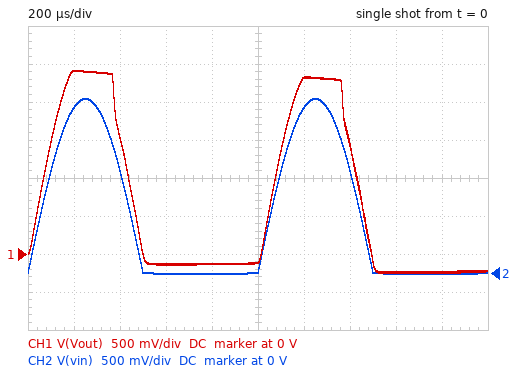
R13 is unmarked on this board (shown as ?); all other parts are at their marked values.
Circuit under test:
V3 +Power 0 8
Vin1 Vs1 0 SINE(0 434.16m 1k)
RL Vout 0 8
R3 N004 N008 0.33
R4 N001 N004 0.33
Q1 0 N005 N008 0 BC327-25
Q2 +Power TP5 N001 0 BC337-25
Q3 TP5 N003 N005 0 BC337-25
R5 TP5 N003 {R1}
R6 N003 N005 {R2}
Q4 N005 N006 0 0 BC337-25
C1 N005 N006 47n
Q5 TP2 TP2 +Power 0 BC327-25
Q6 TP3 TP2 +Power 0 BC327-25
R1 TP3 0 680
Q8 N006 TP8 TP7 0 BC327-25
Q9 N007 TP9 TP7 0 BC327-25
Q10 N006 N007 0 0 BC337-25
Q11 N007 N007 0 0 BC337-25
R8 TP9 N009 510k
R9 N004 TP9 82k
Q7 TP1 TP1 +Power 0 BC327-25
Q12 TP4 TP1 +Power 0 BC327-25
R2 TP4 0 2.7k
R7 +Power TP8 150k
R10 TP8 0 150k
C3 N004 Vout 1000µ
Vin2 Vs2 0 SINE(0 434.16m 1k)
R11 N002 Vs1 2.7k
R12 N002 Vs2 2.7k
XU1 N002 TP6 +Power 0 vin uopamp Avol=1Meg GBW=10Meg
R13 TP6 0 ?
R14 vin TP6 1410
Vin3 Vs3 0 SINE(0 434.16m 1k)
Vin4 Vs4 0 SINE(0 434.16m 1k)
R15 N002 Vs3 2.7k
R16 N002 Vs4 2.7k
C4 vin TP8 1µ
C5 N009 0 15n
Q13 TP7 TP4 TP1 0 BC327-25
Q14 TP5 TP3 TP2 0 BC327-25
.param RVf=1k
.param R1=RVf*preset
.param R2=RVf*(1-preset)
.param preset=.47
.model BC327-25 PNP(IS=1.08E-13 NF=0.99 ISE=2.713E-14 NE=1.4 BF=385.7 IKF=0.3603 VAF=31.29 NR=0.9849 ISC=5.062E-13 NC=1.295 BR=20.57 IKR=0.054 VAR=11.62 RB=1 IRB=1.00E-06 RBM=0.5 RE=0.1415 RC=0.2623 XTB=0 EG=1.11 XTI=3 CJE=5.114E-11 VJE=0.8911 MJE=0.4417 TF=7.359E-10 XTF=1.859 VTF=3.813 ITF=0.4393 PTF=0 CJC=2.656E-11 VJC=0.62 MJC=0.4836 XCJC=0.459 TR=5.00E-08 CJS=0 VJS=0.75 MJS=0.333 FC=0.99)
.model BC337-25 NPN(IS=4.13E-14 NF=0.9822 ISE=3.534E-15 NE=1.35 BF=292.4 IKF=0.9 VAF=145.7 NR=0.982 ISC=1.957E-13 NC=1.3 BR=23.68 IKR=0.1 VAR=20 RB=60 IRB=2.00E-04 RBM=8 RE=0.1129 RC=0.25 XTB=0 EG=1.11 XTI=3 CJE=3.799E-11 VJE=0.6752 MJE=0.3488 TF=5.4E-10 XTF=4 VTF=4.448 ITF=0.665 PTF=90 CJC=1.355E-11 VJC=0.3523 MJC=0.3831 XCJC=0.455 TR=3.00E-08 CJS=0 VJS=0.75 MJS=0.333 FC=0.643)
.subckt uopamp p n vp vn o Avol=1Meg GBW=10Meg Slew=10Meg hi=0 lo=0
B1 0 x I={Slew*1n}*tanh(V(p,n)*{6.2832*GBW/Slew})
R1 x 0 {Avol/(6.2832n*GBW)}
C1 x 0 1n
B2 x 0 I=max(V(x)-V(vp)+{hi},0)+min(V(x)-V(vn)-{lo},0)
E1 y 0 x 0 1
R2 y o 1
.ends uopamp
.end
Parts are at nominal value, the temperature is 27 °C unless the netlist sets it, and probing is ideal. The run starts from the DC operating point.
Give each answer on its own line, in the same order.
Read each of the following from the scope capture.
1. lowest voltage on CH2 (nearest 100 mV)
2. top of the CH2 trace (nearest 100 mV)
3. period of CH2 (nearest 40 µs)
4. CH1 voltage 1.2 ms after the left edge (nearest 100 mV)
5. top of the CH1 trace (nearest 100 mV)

0 V
2.3 V
1.00 ms
2.3 V
2.4 V
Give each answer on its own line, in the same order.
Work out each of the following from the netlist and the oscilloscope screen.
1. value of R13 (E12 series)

330 Ω
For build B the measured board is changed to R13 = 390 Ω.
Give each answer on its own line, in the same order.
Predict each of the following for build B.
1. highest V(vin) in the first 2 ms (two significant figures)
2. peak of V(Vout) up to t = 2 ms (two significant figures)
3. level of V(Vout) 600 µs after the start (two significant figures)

2.0 V
2.3 V
-120 mV
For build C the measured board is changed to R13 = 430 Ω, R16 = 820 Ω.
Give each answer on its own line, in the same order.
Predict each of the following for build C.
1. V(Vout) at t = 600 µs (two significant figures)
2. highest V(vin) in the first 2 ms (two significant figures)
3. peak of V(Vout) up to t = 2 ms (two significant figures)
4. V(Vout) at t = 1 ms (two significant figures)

-110 mV
1.9 V
2.1 V
-98 mV
